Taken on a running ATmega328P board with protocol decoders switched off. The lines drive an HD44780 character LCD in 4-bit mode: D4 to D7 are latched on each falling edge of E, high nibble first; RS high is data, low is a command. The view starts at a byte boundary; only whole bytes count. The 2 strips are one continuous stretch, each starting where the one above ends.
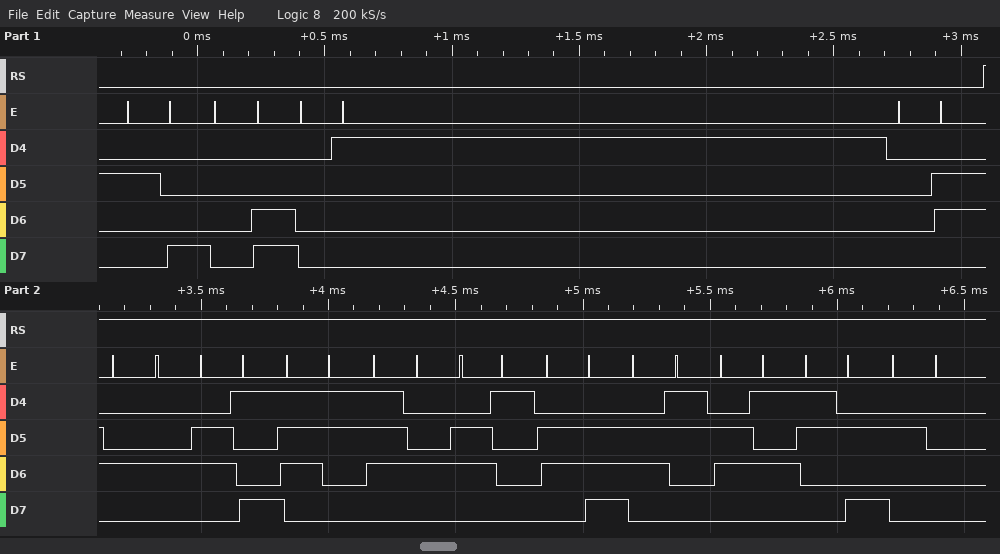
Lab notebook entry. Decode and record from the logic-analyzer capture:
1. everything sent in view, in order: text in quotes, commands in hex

0x28 0x0C 0x01 0x06 "Distance: "
